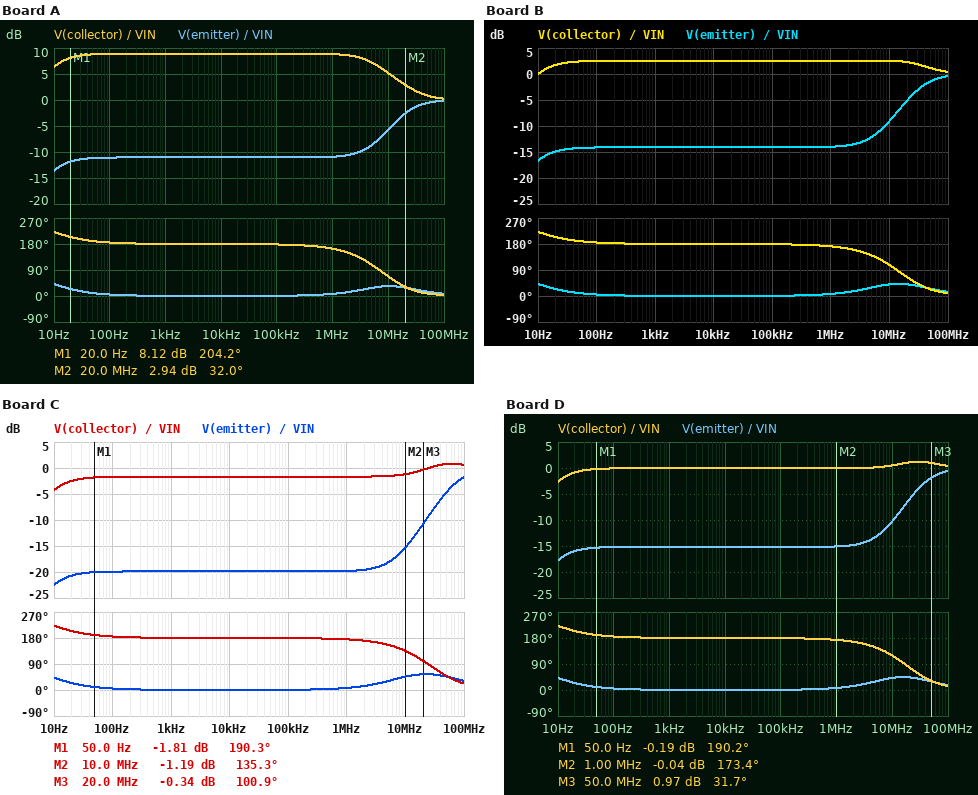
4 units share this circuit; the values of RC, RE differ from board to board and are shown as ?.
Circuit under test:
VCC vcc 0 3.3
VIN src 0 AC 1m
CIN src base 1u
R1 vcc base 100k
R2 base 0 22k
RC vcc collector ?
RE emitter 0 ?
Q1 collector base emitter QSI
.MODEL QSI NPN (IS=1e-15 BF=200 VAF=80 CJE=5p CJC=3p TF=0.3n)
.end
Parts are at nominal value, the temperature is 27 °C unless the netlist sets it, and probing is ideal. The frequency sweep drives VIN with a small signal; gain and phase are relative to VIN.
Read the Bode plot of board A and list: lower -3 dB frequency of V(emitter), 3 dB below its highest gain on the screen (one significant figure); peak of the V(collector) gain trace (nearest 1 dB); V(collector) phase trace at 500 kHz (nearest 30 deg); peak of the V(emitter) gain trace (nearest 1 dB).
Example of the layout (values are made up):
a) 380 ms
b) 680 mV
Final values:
a) 20 MHz
b) 9 dB
c) 180 deg
d) 0 dB
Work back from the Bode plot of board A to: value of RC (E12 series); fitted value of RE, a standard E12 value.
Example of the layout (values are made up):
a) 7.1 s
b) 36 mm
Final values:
a) 15 kΩ
b) 1.5 kΩ
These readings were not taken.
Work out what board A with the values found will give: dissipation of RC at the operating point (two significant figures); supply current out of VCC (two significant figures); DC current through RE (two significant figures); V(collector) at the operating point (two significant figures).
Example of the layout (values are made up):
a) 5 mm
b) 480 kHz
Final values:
a) 670 nW
b) 34 µA
c) 6.7 µA
d) 3.2 V
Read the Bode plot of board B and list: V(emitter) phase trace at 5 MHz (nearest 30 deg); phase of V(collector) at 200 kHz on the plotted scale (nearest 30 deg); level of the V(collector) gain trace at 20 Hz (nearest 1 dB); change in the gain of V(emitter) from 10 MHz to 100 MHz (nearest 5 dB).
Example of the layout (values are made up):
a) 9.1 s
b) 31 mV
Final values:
a) 30 deg
b) 180 deg
c) 2 dB
d) 10 dB
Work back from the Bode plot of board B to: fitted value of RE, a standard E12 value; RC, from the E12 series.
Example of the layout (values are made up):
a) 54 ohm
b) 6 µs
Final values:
a) 820 Ω
b) 5.6 kΩ
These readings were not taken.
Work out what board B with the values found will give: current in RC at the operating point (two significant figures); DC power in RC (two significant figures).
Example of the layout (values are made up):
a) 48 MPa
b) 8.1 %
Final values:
a) 7.7 µA
b) 330 nW
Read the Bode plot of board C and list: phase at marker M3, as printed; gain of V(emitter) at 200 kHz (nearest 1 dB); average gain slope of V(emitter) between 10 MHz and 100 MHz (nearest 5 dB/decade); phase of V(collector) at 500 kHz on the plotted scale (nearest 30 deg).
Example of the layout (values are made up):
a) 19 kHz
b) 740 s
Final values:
a) 100.9 deg
b) -20 dB
c) 15 dB/decade
d) 180 deg
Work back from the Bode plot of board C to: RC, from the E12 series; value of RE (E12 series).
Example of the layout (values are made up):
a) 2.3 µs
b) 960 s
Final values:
a) 2.7 kΩ
b) 330 Ω
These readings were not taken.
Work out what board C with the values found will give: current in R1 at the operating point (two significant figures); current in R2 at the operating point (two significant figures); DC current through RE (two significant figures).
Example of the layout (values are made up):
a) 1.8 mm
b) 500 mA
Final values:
a) 27 µA
b) 27 µA
c) 8.8 µA
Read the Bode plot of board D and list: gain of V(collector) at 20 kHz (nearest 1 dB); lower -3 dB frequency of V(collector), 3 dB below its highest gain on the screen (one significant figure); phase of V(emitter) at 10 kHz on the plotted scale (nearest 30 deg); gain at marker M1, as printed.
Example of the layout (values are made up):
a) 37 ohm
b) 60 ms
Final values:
a) 0 dB
b) 10 Hz
c) 0 deg
d) -0.19 dB
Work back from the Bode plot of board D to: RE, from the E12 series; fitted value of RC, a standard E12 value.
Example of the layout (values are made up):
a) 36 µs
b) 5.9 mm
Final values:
a) 680 Ω
b) 3.9 kΩ
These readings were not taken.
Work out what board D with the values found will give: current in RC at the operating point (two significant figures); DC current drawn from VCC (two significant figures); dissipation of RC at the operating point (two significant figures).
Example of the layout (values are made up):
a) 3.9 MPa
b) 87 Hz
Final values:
a) 8.0 µA
b) 35 µA
c) 250 nW
